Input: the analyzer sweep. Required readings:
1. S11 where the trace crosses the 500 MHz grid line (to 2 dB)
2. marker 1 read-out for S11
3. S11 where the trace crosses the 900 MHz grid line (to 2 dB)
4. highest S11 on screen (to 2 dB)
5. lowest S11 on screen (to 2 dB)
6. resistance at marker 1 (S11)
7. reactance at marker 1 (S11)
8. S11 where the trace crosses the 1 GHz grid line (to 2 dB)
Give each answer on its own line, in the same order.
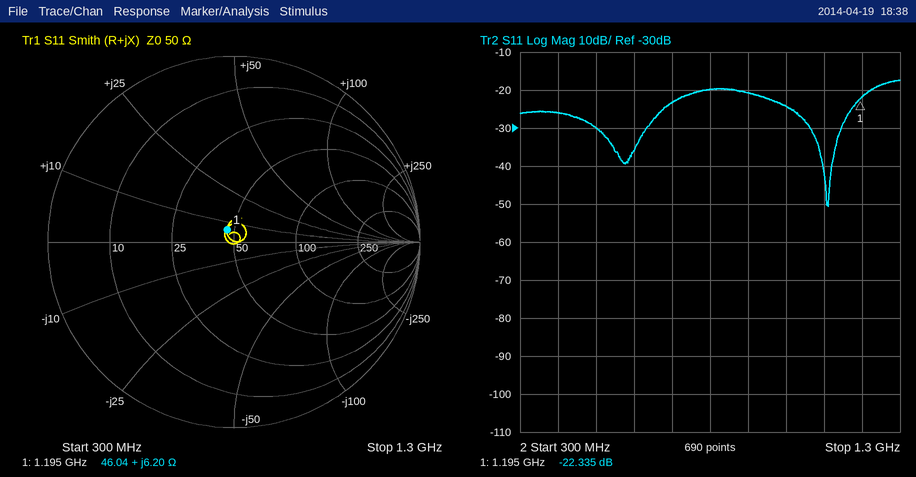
-30 dB
-22.335 dB
-20 dB
-18 dB
-50 dB
46.04 Ω
+6.20 Ω
-24 dB
